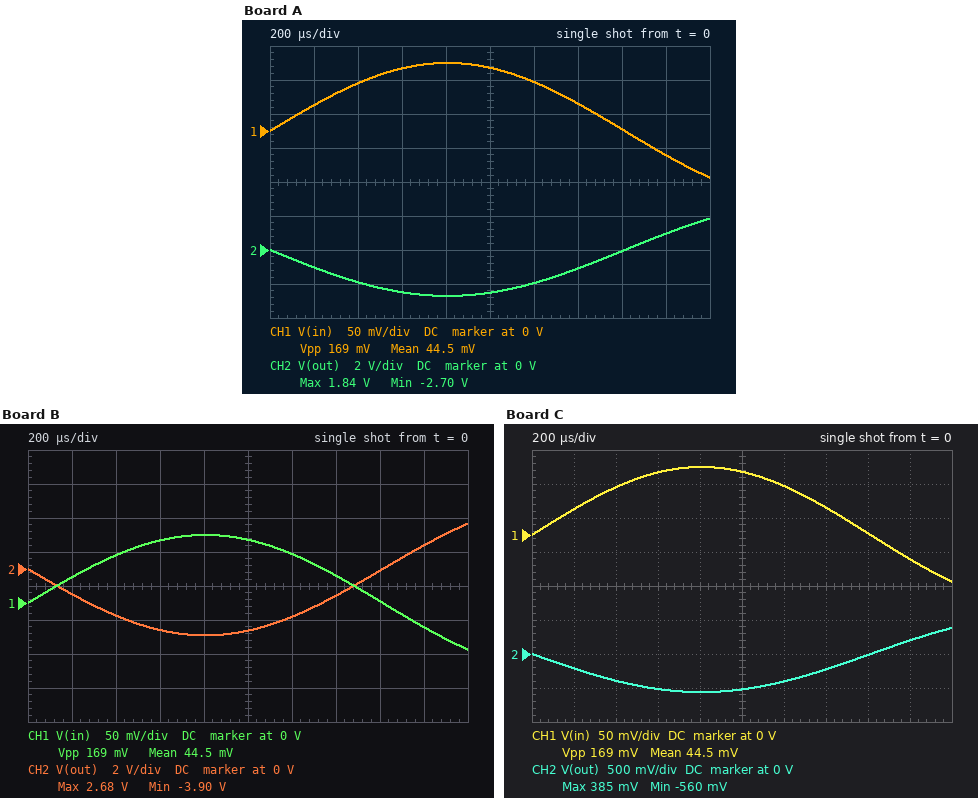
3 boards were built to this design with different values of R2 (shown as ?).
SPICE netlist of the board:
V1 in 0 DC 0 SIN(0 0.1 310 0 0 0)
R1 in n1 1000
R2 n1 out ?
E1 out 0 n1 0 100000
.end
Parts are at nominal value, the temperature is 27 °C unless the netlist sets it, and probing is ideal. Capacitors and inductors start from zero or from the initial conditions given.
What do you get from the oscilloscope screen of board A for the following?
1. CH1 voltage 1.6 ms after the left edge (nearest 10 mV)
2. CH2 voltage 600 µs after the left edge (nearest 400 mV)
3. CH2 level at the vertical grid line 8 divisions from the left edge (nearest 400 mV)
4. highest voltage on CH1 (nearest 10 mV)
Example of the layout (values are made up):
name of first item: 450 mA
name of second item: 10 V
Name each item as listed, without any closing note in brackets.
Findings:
CH1 voltage 1.6 ms after the left edge: 0 V
CH2 voltage 600 µs after the left edge: -2.4 V
CH2 level at the vertical grid line 8 divisions from the left edge: 0 V
highest voltage on CH1: 100 mV
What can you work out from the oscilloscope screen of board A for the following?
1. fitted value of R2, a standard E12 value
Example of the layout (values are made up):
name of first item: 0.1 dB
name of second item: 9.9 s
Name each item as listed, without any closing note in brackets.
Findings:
fitted value of R2, a standard E12 value: 27 kΩ
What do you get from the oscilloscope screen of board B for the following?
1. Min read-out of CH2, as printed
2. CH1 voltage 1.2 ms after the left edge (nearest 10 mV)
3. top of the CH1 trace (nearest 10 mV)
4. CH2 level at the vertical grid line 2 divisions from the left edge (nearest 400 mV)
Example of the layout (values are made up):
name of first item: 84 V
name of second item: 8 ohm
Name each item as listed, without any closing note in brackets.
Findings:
Min read-out of CH2, as printed: -3.90 V
CH1 voltage 1.2 ms after the left edge: 70 mV
top of the CH1 trace: 100 mV
CH2 level at the vertical grid line 2 divisions from the left edge: -2.8 V
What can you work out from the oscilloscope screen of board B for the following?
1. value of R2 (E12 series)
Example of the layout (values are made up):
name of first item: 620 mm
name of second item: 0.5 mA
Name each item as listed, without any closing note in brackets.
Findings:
value of R2: 39 kΩ
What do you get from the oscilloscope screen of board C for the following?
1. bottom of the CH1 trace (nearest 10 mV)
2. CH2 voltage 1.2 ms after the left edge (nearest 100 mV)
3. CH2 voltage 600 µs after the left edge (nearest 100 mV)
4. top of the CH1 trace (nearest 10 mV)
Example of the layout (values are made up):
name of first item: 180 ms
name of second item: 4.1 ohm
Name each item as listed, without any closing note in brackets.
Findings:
bottom of the CH1 trace: -70 mV
CH2 voltage 1.2 ms after the left edge: -400 mV
CH2 voltage 600 µs after the left edge: -500 mV
top of the CH1 trace: 100 mV
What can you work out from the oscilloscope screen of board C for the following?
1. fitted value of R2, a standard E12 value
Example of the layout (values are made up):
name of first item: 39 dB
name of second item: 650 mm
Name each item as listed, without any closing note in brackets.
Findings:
fitted value of R2, a standard E12 value: 5.6 kΩ
